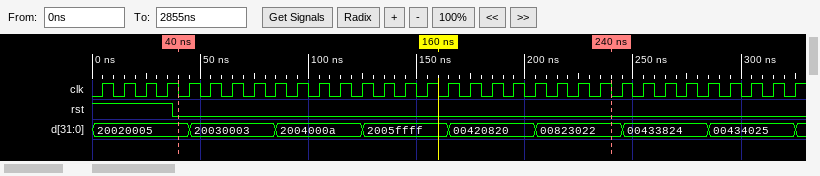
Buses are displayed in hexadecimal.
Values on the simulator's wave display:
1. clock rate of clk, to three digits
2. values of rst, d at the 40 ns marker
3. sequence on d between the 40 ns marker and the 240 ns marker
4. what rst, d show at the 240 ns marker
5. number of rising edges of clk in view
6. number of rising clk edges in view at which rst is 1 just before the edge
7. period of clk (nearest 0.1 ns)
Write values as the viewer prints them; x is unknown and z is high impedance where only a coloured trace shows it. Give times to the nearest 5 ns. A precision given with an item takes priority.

100 MHz
rst=0, d=20020005
20020005, 20030003, 2004000a, 2005ffff, 00420820, 00823022
rst=0, d=00823022
33
4
10 ns
